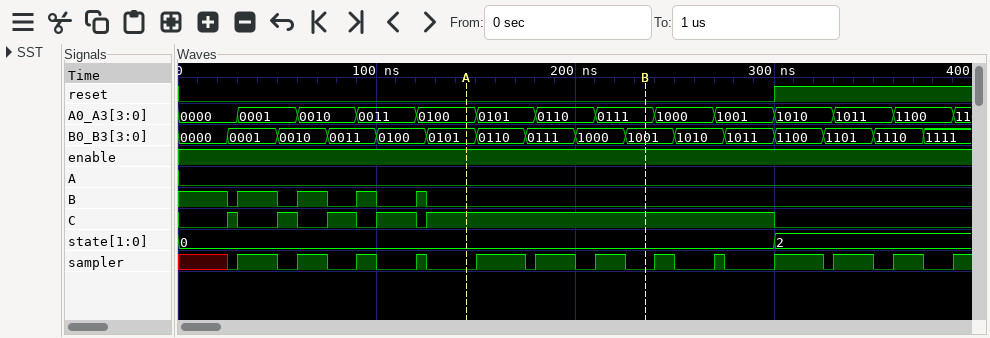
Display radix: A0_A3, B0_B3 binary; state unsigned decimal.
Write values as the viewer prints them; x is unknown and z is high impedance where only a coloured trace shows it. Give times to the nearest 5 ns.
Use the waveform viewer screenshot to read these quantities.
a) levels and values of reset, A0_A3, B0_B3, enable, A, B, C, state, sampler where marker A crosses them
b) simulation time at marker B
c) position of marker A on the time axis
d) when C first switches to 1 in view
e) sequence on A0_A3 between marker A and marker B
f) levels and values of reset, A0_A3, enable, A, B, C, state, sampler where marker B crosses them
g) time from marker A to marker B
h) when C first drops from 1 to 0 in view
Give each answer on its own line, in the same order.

reset=0, A0_A3=0100, B0_B3=0101, enable=1, A=0, B=0, C=1, state=0, sampler=0
235 ns
145 ns
25 ns
0100, 0101, 0110, 0111
reset=0, A0_A3=0111, enable=1, A=0, B=0, C=1, state=0, sampler=0
90 ns
30 ns
